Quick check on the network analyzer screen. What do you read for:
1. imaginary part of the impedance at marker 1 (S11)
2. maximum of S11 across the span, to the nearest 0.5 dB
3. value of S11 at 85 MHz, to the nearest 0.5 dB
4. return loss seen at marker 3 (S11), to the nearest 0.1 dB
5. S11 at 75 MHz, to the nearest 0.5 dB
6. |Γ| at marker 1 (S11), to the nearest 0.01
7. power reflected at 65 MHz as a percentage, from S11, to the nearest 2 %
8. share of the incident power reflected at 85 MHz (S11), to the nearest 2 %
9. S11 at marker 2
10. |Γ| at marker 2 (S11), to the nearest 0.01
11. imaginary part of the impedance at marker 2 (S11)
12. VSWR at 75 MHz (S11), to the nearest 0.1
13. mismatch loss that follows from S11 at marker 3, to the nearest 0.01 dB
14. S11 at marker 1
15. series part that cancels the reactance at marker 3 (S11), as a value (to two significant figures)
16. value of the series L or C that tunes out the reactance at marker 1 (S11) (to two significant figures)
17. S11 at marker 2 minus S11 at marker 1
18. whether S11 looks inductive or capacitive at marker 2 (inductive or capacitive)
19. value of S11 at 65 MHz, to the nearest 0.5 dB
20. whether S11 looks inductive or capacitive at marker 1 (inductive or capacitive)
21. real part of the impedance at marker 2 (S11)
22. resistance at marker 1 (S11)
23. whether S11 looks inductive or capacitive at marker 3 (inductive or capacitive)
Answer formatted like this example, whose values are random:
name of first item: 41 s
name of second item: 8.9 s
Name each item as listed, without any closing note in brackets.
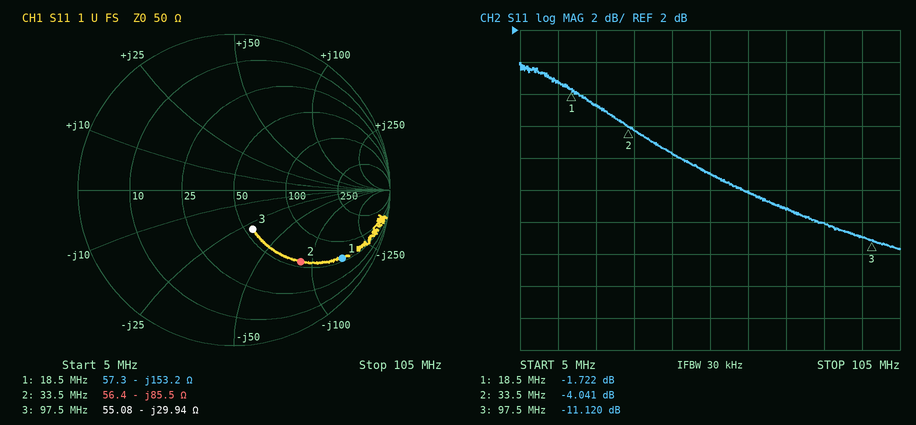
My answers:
imaginary part of the impedance at marker 1: -153.2 Ω
maximum of S11 across the span, to the nearest 0.5 dB: 0.0 dB
value of S11 at 85 MHz, to the nearest 0.5 dB: -10.0 dB
return loss seen at marker 3 (S11), to the nearest 0.1 dB: 11.1 dB
S11 at 75 MHz, to the nearest 0.5 dB: -9.0 dB
|Γ| at marker 1 (S11), to the nearest 0.01: 0.82
power reflected at 65 MHz as a percentage, from S11, to the nearest 2 %: 16 %
share of the incident power reflected at 85 MHz (S11), to the nearest 2 %: 10 %
S11 at marker 2: -4.041 dB
|Γ| at marker 2 (S11), to the nearest 0.01: 0.63
imaginary part of the impedance at marker 2: -85.5 Ω
VSWR at 75 MHz (S11), to the nearest 0.1: 2.1
mismatch loss that follows from S11 at marker 3, to the nearest 0.01 dB: 0.35 dB
S11 at marker 1: -1.722 dB
series part that cancels the reactance at marker 3 (S11), as a value: 49 nH
value of the series L or C that tunes out the reactance at marker 1 (S11): 1.3 µH
S11 at marker 2 minus S11 at marker 1: -2.319 dB
whether S11 looks inductive or capacitive at marker 2: capacitive
value of S11 at 65 MHz, to the nearest 0.5 dB: -8.0 dB
whether S11 looks inductive or capacitive at marker 1: capacitive
real part of the impedance at marker 2: 56.4 Ω
resistance at marker 1: 57.3 Ω
whether S11 looks inductive or capacitive at marker 3: capacitive
